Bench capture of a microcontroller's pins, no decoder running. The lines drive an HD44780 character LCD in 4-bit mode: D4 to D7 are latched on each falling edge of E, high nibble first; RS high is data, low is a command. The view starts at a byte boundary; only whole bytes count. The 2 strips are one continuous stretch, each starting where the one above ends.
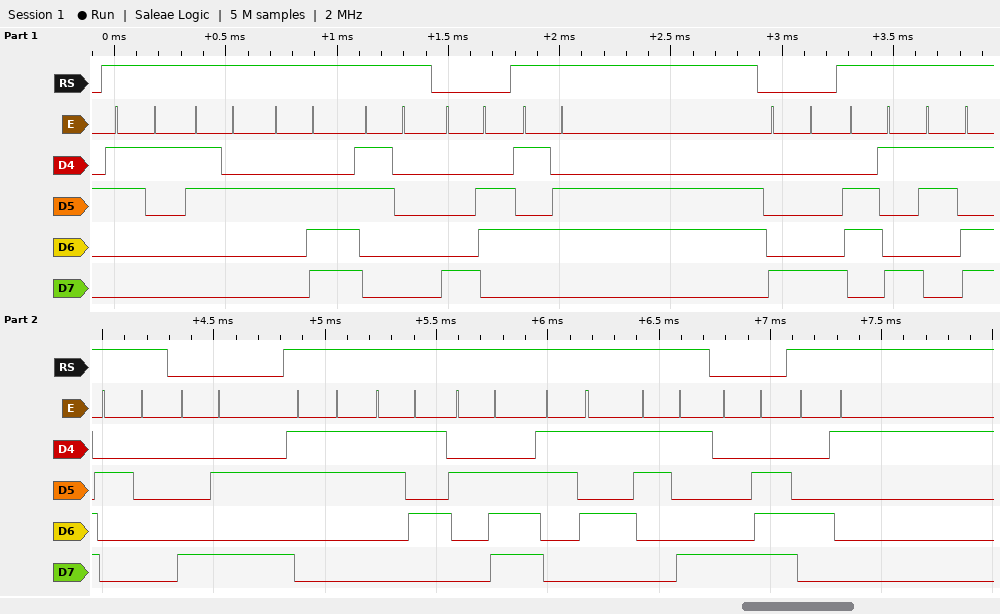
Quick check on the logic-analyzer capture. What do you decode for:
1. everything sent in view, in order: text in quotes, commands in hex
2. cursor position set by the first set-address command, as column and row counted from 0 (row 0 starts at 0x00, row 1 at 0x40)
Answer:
"12.0" 0x86 "V" 0x88 "i= " 0x8A "35.59" 0x8E "A"
column 6, row 0
